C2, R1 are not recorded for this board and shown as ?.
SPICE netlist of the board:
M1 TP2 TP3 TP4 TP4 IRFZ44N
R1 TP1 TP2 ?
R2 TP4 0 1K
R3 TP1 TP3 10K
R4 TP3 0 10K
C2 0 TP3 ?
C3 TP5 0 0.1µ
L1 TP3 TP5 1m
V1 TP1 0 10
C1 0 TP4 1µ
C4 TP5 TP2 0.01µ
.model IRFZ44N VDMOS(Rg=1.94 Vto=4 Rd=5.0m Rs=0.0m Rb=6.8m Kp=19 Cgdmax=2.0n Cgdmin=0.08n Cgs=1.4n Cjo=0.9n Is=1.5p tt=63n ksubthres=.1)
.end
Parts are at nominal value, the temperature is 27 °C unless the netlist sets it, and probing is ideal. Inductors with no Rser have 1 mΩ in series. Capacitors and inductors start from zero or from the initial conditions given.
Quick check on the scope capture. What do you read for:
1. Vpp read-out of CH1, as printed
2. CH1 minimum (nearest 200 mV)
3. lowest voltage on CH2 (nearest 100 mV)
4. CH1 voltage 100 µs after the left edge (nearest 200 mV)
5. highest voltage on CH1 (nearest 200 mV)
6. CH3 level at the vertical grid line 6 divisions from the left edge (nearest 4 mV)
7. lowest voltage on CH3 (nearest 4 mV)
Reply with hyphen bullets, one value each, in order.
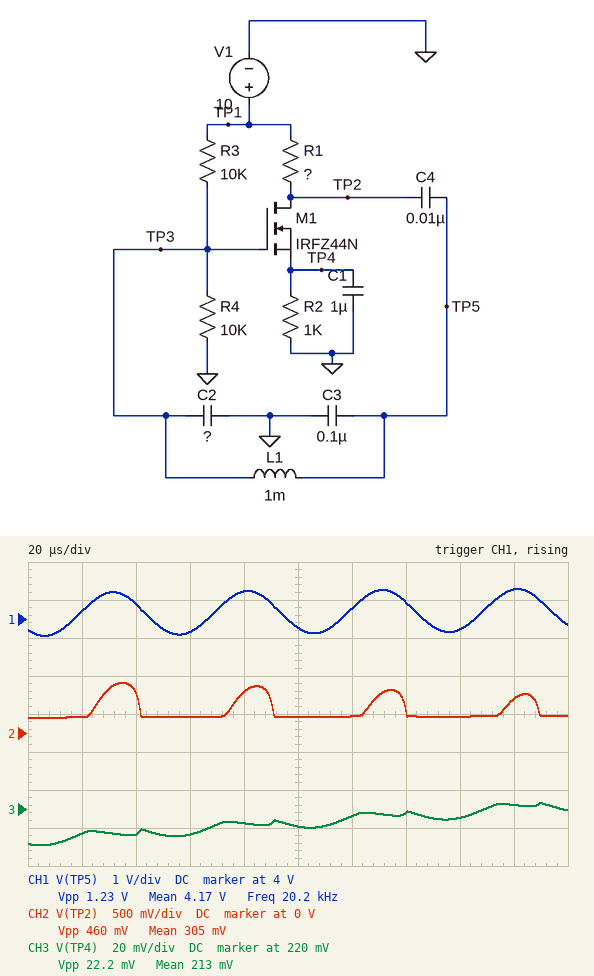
- 1.23 V
- 3.6 V
- 200 mV
- 3.8 V
- 4.8 V
- 216 mV
- 200 mV
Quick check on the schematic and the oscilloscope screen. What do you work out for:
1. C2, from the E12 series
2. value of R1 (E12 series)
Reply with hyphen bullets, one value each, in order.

- 150 nF
- 33 kΩ
